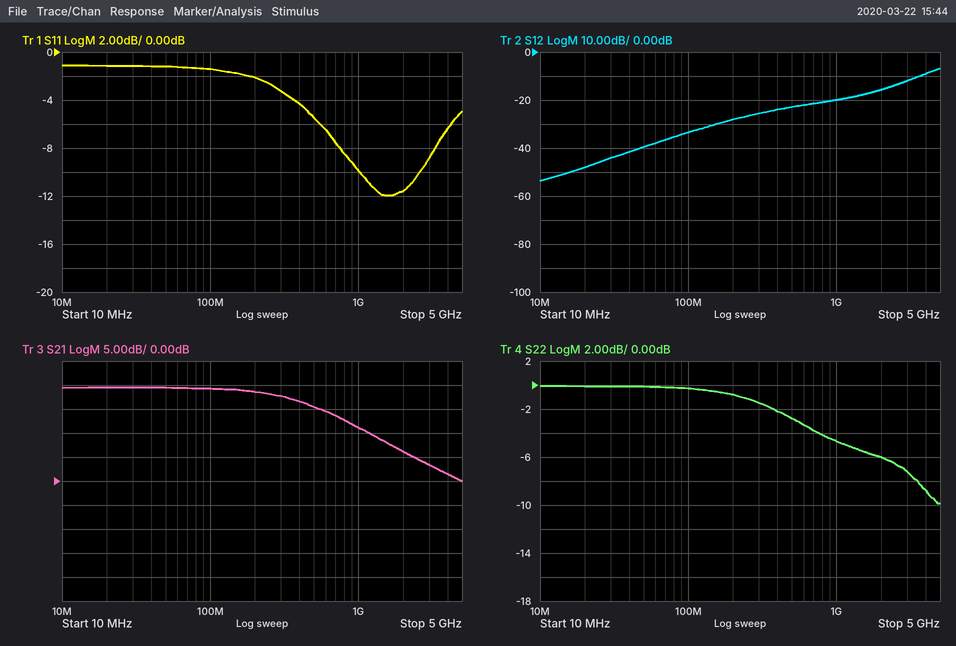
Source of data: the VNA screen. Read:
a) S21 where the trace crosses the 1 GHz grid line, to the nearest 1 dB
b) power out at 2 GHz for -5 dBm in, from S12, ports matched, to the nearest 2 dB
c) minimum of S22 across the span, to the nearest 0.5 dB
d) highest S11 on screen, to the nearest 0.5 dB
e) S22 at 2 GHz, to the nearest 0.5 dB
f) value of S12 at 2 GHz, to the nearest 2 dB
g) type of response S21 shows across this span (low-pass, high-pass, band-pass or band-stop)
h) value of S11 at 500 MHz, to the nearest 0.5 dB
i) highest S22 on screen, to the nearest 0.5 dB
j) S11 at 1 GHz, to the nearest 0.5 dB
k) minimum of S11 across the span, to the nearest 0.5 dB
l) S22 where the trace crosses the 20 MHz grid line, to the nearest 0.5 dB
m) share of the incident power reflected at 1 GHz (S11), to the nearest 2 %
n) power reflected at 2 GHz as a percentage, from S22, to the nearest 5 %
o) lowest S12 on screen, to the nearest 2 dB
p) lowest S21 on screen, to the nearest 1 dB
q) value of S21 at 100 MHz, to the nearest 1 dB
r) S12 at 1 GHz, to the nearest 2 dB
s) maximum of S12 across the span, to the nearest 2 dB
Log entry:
11 dB
-20 dBm
-10.0 dB
-1.0 dB
-6.0 dB
-16 dB
low-pass
-5.5 dB
0.0 dB
-10.0 dB
-12.0 dB
0.0 dB
10 %
25 %
-54 dB
0 dB
19 dB
-20 dB
-6 dB
